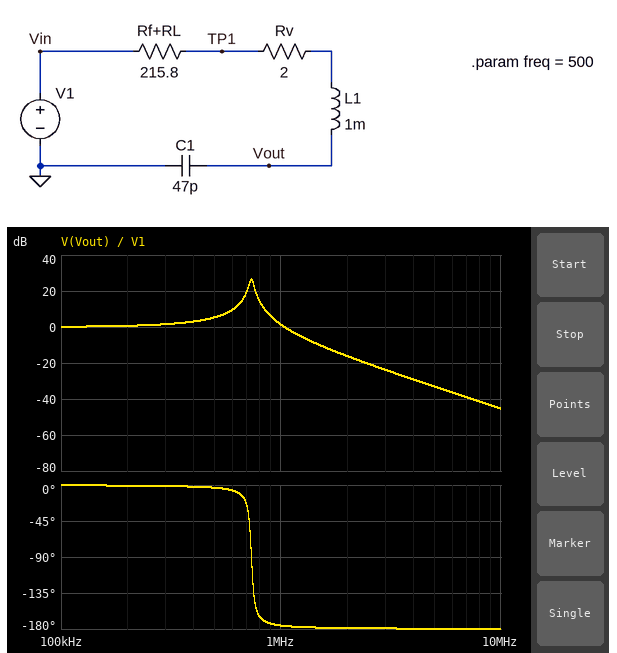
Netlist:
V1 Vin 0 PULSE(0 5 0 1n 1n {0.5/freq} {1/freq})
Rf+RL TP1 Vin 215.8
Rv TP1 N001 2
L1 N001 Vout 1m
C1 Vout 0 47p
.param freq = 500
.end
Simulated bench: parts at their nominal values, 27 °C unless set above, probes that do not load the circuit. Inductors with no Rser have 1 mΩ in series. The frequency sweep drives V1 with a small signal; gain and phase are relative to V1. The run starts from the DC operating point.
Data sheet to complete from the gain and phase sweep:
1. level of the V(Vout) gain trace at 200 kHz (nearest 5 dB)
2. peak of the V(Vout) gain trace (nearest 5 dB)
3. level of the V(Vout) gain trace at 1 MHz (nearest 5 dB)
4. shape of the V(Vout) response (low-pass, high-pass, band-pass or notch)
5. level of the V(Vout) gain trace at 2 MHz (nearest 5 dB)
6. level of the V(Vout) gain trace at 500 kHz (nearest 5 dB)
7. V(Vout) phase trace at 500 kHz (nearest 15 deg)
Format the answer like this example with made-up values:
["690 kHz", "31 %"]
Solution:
["0 dB", "25 dB", "0 dB", "low-pass", "-15 dB", "5 dB", "0 deg"]
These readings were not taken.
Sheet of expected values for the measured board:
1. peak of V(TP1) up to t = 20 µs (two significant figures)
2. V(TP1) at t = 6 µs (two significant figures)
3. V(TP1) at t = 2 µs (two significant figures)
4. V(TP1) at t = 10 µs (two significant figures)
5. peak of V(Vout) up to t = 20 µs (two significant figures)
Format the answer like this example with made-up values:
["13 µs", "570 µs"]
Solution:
["5.2 V", "4.9 V", "5.0 V", "4.9 V", "9.6 V"]
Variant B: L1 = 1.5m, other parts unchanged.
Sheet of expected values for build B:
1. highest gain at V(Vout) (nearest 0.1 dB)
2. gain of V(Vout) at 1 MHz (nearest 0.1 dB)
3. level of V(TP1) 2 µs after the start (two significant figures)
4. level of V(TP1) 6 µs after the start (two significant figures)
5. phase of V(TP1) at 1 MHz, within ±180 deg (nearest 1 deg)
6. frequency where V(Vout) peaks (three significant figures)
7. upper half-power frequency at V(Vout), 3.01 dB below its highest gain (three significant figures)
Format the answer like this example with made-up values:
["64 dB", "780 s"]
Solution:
["28.3 dB", "-5.0 dB", "4.8 V", "5.1 V", "2 deg", "599 kHz", "611 kHz"]
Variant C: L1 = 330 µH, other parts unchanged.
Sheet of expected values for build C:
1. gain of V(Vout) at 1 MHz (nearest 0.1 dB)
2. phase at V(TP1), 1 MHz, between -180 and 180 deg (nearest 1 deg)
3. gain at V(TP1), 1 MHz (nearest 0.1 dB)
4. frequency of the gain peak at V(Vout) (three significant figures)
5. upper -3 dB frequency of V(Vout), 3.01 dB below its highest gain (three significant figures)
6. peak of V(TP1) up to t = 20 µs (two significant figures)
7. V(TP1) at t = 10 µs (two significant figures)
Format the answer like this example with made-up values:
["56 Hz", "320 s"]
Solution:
["8.1 dB", "-9 deg", "-0.1 dB", "1.28 MHz", "1.33 MHz", "5.3 V", "5.0 V"]
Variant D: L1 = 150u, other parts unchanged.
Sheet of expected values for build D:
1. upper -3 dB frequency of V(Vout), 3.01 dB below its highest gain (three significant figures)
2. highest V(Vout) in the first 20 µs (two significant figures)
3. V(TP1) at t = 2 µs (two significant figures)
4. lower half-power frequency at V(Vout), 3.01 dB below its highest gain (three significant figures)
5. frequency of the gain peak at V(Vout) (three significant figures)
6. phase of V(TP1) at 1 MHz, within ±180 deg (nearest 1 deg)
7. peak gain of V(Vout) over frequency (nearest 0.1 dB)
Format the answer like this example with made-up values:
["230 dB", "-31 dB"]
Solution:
["2.00 MHz", "9.1 V", "5.1 V", "1.77 MHz", "1.89 MHz", "-5 deg", "18.3 dB"]
